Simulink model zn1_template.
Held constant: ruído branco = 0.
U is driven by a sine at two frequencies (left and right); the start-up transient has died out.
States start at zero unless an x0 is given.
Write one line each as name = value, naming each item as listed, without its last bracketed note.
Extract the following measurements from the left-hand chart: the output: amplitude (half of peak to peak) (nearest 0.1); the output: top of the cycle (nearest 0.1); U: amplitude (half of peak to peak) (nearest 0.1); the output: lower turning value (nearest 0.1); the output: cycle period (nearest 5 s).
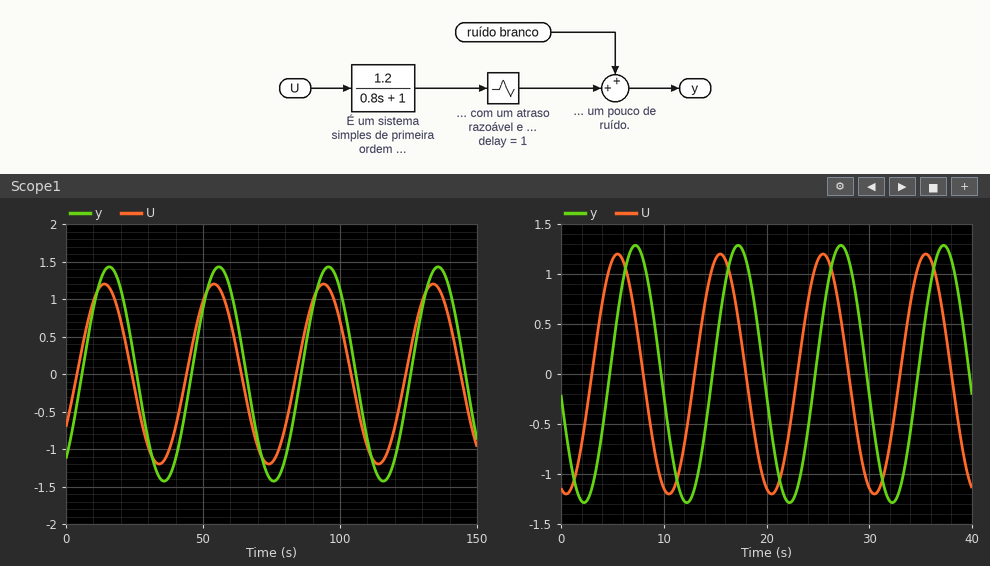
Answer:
the output: amplitude (half of peak to peak) = 1.4
the output: top of the cycle = 1.4
U: amplitude (half of peak to peak) = 1.2
the output: lower turning value = -1.4
the output: cycle period = 40 s
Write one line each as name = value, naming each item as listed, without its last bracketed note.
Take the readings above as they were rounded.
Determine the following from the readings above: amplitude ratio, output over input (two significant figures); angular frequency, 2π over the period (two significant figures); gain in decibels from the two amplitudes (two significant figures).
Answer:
amplitude ratio, output over input = 1.2
angular frequency, 2π over the period = 0.16 rad/s
gain in decibels from the two amplitudes = 1.3 dB
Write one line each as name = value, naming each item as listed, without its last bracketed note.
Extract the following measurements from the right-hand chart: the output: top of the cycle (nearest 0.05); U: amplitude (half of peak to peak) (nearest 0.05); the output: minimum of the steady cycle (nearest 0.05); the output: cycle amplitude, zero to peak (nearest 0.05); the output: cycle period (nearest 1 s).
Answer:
the output: top of the cycle = 1.30
U: amplitude (half of peak to peak) = 1.20
the output: minimum of the steady cycle = -1.30
the output: cycle amplitude, zero to peak = 1.30
the output: cycle period = 10 s
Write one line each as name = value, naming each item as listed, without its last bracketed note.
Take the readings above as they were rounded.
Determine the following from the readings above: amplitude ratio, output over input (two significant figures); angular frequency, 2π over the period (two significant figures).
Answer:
amplitude ratio, output over input = 1.1
angular frequency, 2π over the period = 0.63 rad/s
